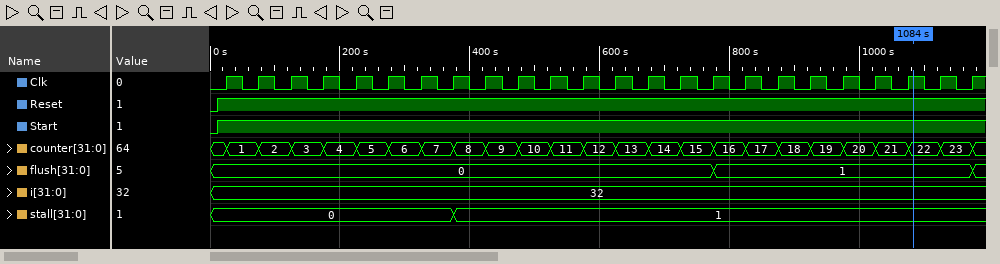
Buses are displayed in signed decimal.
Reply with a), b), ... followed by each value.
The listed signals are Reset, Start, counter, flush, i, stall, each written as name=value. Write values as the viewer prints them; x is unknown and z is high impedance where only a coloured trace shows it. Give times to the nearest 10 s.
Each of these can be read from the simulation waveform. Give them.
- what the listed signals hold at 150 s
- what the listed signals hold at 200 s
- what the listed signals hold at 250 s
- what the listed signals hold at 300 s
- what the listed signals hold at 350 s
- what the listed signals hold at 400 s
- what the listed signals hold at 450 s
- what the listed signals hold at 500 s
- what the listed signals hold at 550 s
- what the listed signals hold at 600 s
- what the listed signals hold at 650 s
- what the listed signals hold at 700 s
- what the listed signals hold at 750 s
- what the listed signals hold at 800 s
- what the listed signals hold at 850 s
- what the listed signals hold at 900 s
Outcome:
a) Reset=1, Start=1, counter=3, flush=0, i=32, stall=0
b) Reset=1, Start=1, counter=4, flush=0, i=32, stall=0
c) Reset=1, Start=1, counter=5, flush=0, i=32, stall=0
d) Reset=1, Start=1, counter=6, flush=0, i=32, stall=0
e) Reset=1, Start=1, counter=7, flush=0, i=32, stall=0
f) Reset=1, Start=1, counter=8, flush=0, i=32, stall=1
g) Reset=1, Start=1, counter=9, flush=0, i=32, stall=1
h) Reset=1, Start=1, counter=10, flush=0, i=32, stall=1
i) Reset=1, Start=1, counter=11, flush=0, i=32, stall=1
j) Reset=1, Start=1, counter=12, flush=0, i=32, stall=1
k) Reset=1, Start=1, counter=13, flush=0, i=32, stall=1
l) Reset=1, Start=1, counter=14, flush=0, i=32, stall=1
m) Reset=1, Start=1, counter=15, flush=0, i=32, stall=1
n) Reset=1, Start=1, counter=16, flush=1, i=32, stall=1
o) Reset=1, Start=1, counter=17, flush=1, i=32, stall=1
p) Reset=1, Start=1, counter=18, flush=1, i=32, stall=1
